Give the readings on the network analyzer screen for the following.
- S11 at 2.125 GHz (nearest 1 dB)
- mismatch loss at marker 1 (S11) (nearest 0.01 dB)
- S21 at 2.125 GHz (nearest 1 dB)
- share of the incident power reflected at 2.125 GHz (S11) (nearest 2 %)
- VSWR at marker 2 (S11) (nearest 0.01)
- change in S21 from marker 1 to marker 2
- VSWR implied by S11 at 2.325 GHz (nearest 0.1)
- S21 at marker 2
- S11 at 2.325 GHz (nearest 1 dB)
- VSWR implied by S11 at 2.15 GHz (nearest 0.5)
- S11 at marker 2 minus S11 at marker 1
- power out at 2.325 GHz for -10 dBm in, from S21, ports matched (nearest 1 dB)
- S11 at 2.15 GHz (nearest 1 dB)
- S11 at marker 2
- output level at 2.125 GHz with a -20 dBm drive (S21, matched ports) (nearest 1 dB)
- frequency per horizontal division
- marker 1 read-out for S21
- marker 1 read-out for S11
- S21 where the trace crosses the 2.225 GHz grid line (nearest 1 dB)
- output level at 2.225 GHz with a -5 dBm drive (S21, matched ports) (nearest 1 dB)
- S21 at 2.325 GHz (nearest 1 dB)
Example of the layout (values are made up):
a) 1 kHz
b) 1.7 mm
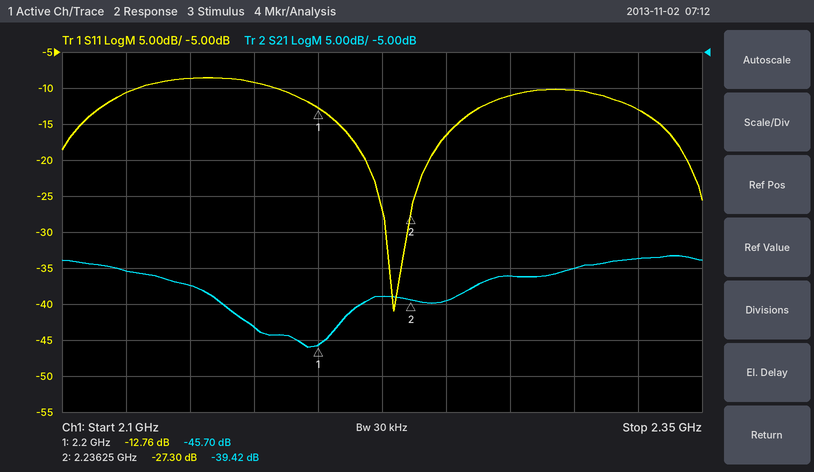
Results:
a) -11 dB
b) 0.24 dB
c) -35 dB
d) 8 %
e) 1.09
f) 6.28 dB
g) 1.6
h) -39.42 dB
i) -13 dB
j) 2.0
k) -14.54 dB
l) -44 dBm
m) -9 dB
n) -27.30 dB
o) -55 dBm
p) 25 MHz
q) -45.70 dB
r) -12.76 dB
s) -39 dB
t) -44 dBm
u) -34 dB
